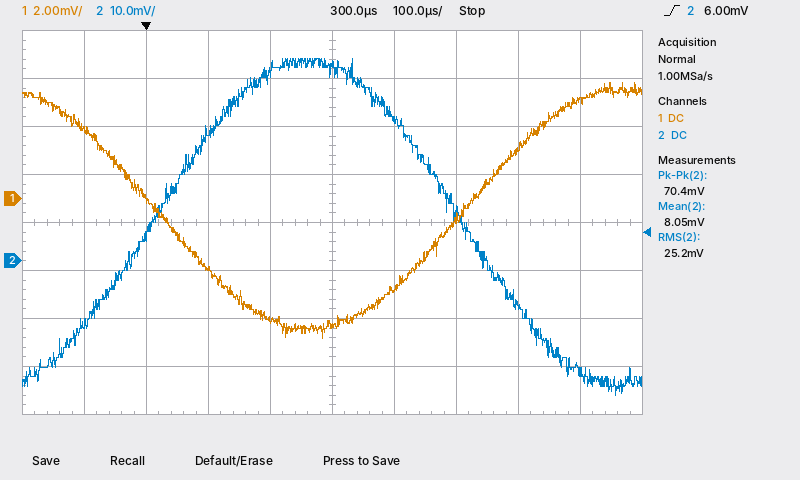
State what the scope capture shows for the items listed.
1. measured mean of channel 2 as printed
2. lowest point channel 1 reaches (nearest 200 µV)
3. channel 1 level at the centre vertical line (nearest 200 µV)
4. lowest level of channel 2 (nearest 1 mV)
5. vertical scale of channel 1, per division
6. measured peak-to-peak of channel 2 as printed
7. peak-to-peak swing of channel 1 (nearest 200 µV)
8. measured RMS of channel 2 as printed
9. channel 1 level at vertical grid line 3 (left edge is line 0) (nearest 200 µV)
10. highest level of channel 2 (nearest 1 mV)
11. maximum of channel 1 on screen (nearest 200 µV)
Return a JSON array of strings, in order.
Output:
["8.05 mV", "-5.8 mV", "-5.2 mV", "-28 mV", "2 mV", "70.4 mV", "10.6 mV", "25.2 mV", "-3.0 mV", "42 mV", "4.8 mV"]
